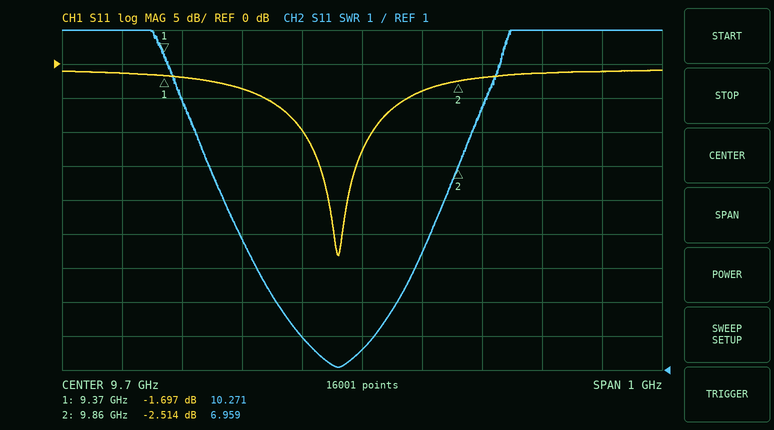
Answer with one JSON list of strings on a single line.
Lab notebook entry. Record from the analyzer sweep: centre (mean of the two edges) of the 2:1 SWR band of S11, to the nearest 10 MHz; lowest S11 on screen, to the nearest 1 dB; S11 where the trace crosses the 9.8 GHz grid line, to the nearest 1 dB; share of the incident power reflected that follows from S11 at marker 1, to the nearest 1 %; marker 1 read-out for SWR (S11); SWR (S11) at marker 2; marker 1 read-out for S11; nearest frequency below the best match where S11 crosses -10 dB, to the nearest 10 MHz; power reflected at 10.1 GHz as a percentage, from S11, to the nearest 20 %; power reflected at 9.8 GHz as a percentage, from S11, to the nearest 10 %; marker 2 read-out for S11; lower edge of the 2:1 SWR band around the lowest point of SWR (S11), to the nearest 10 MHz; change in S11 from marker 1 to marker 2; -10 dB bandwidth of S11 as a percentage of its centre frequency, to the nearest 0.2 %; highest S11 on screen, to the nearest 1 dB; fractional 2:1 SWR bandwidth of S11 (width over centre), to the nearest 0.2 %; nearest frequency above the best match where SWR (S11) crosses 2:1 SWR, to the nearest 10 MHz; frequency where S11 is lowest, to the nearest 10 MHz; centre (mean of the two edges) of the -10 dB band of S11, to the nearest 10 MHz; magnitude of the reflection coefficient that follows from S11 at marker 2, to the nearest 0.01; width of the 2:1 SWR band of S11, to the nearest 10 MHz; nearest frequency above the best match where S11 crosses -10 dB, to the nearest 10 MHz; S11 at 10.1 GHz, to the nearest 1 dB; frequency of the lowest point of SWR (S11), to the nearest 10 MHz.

["9.66 GHz", "-28 dB", "-4 dB", "68 %", "10.271", "6.959", "-1.697 dB", "9.60 GHz", "80 %", "40 %", "-2.514 dB", "9.60 GHz", "-0.817 dB", "1.2 %", "-1 dB", "1.2 %", "9.72 GHz", "9.66 GHz", "9.66 GHz", "0.75", "120 MHz", "9.72 GHz", "-1 dB", "9.66 GHz"]
